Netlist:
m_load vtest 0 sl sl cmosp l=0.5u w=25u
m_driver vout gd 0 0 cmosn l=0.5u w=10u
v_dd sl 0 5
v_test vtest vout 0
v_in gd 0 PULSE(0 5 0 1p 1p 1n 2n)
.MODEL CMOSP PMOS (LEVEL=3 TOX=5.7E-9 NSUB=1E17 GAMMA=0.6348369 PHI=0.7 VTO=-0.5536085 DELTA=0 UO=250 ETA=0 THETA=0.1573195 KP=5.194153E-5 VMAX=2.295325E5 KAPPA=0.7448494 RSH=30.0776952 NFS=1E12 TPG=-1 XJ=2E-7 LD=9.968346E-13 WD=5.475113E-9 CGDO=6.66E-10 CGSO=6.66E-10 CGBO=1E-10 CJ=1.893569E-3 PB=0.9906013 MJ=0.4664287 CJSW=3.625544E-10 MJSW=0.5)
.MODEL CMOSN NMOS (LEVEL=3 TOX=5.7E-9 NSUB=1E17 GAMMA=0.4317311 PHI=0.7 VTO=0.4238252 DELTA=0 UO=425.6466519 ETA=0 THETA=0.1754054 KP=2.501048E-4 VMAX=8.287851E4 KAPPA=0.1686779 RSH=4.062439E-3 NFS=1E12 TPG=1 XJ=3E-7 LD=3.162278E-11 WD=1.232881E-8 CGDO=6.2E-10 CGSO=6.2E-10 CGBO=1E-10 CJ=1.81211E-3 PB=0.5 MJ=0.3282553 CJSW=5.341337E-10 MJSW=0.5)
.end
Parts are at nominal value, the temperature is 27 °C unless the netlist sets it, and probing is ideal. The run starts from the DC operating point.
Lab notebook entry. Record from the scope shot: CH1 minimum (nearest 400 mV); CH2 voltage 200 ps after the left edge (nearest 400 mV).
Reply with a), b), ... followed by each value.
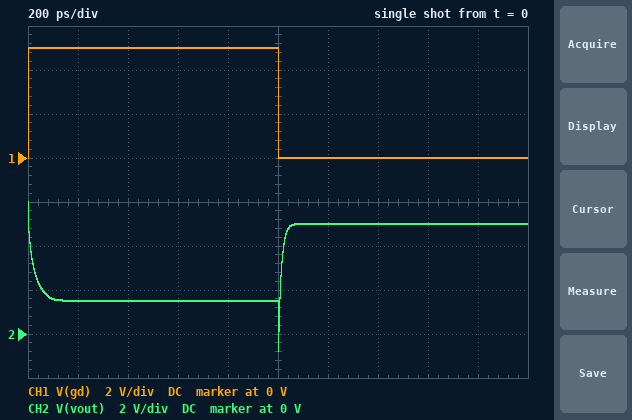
a) 0 V
b) 1.6 V
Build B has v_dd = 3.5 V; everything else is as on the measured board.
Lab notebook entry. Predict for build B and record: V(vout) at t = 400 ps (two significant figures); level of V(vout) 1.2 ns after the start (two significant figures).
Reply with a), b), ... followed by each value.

a) 520 mV
b) 3.5 V
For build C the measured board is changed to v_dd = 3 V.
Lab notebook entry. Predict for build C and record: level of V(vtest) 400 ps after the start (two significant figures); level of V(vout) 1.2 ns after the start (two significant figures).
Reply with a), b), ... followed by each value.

a) 360 mV
b) 3.0 V
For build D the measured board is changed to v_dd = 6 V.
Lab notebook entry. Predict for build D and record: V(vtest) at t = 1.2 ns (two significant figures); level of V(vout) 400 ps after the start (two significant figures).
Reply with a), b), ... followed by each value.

a) 6.0 V
b) 3.4 V
